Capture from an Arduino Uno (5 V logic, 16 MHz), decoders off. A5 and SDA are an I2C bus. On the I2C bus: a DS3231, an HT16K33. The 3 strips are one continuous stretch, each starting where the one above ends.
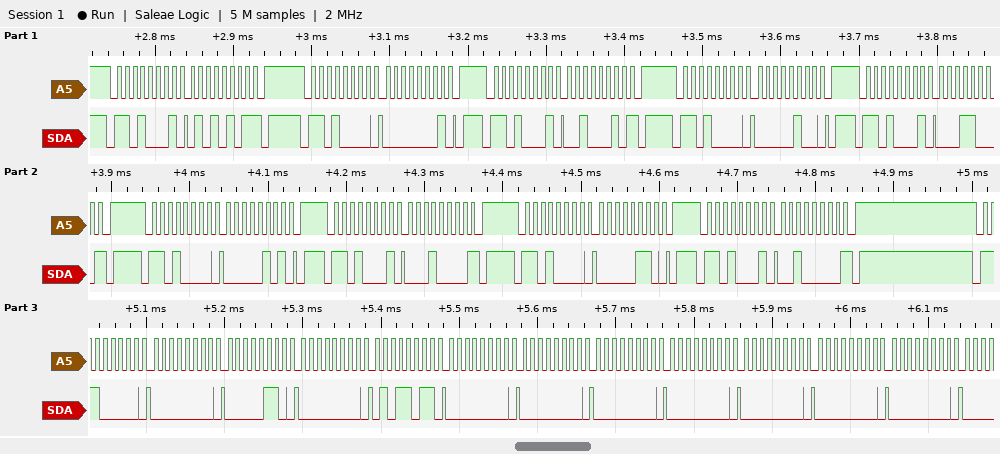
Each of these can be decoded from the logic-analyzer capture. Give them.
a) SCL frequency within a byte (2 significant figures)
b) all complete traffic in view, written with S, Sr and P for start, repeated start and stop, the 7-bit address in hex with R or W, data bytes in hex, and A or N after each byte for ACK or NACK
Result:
100 kHz
S 68R A 55 N P S 68W A 01 A P S 68R A 22 N P S 68W A 04 A P S 68R A 18 N P S 68W A 05 A P S 68R A 10 N P S 68W A 06 A P S 68R A 20 N P S 70W A 00 A 06 A 00 A 5B A 00 A 00 A 00 A 00 A 00 A 00 A 00 A
